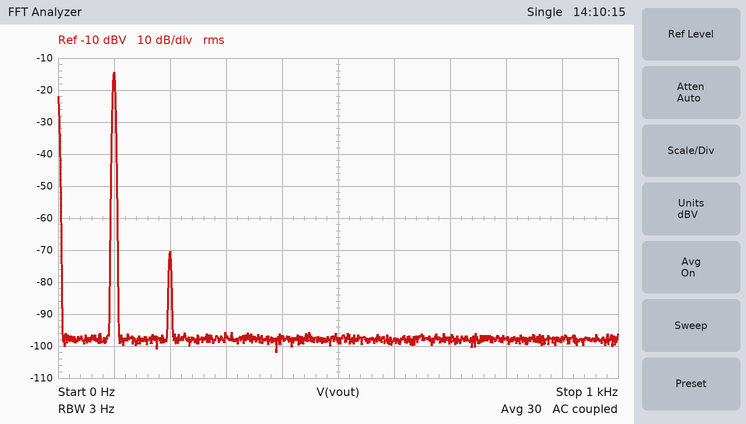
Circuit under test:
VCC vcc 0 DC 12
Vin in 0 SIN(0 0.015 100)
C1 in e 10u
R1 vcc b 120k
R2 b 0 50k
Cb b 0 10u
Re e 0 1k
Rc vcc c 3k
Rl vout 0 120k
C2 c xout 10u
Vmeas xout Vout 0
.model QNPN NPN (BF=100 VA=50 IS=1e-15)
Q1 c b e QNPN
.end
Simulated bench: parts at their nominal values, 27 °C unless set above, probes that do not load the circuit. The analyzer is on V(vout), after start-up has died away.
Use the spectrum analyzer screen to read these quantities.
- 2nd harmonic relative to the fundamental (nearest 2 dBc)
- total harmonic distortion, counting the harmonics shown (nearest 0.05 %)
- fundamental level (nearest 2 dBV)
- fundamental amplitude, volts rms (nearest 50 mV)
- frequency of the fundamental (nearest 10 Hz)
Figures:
-56 dBc
0.15 %
-14 dBV
200 mV
100 Hz
